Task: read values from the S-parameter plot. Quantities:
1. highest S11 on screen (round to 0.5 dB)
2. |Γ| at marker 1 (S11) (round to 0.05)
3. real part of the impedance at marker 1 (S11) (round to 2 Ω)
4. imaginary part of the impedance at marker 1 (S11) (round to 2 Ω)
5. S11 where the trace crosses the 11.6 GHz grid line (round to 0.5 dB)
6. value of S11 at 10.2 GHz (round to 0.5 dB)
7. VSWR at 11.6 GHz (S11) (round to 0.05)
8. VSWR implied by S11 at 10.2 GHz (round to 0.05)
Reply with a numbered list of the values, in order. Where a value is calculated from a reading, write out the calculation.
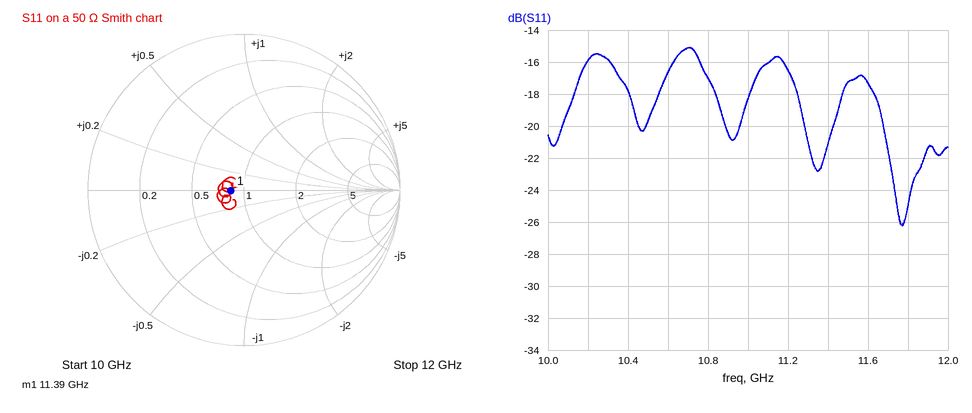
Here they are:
1. -15.0 dB
2. 0.10
3. 42 Ω
4. 0 Ω
5. -17.5 dB
6. -16.0 dB
7. |Γ| = 10^(-17.5/20) = 0.1334; VSWR = (1 + 0.1334)/(1 − 0.1334) ≈ 1.31, so 1.30 to the nearest 0.05
8. |Γ| = 10^(-16/20) = 0.1585; VSWR = (1 + 0.1585)/(1 − 0.1585) ≈ 1.38, so 1.40 to the nearest 0.05
